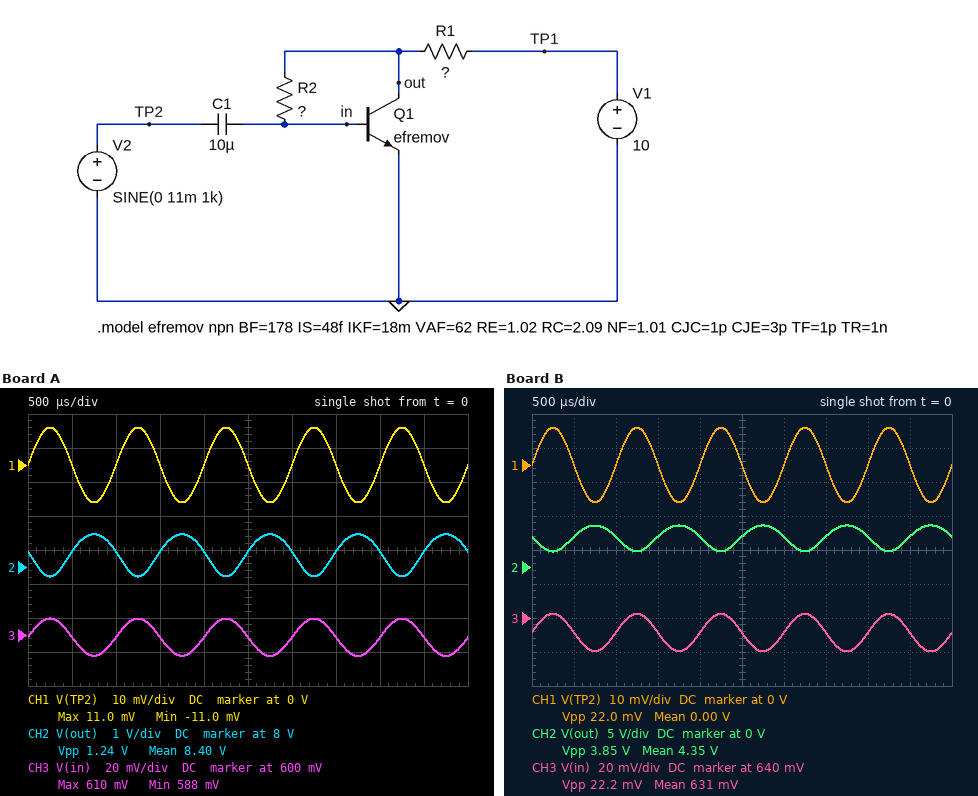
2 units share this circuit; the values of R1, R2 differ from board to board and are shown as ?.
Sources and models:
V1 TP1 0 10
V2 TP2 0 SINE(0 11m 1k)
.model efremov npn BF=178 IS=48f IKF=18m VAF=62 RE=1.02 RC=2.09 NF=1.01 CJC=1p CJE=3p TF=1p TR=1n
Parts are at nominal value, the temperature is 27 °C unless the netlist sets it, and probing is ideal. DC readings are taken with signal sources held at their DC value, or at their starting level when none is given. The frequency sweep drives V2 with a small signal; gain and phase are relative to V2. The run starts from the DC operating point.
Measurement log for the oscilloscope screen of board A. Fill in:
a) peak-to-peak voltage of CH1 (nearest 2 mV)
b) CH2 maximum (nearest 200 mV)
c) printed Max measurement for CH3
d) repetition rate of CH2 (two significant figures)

22 mV
9.0 V
610 mV
1.0 kHz
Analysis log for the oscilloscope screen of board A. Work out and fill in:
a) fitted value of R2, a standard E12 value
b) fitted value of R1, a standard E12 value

3.3 MΩ
3.3 kΩ
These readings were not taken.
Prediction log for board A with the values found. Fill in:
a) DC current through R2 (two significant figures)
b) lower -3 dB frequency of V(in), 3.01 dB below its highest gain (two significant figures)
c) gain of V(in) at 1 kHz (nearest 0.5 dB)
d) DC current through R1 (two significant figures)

2.4 µA
1.7 Hz
0 dB
470 µA
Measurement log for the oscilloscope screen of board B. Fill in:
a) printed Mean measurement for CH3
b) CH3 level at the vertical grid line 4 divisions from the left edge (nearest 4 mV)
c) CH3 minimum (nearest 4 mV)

631 mV
632 mV
620 mV
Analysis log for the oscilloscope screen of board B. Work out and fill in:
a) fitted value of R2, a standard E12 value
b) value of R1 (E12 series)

470 kΩ
3.9 kΩ
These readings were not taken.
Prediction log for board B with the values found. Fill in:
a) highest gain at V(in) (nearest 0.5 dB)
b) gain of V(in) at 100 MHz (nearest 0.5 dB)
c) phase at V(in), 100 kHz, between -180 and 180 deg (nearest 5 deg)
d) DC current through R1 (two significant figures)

0 dB
0 dB
0 deg
1.4 mA
